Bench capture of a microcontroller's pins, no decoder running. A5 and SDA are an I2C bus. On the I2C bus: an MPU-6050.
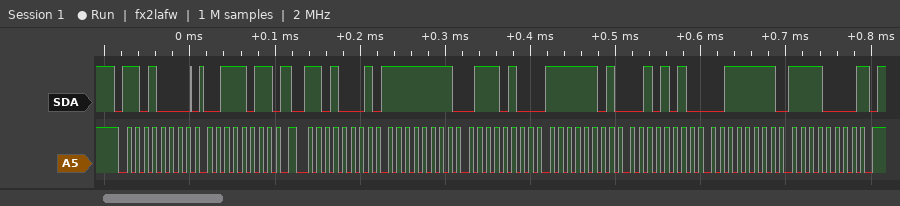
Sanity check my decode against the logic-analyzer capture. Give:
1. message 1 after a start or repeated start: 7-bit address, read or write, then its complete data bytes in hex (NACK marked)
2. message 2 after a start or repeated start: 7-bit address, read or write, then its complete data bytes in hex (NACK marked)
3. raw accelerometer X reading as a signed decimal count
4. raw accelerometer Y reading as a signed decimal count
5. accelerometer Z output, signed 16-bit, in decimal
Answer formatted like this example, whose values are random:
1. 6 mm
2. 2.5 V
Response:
1. 0x68 write: 3B
2. 0x68 read: FF 74 FD 2A 3F F0 NACK
3. -140
4. -726
5. 16368
